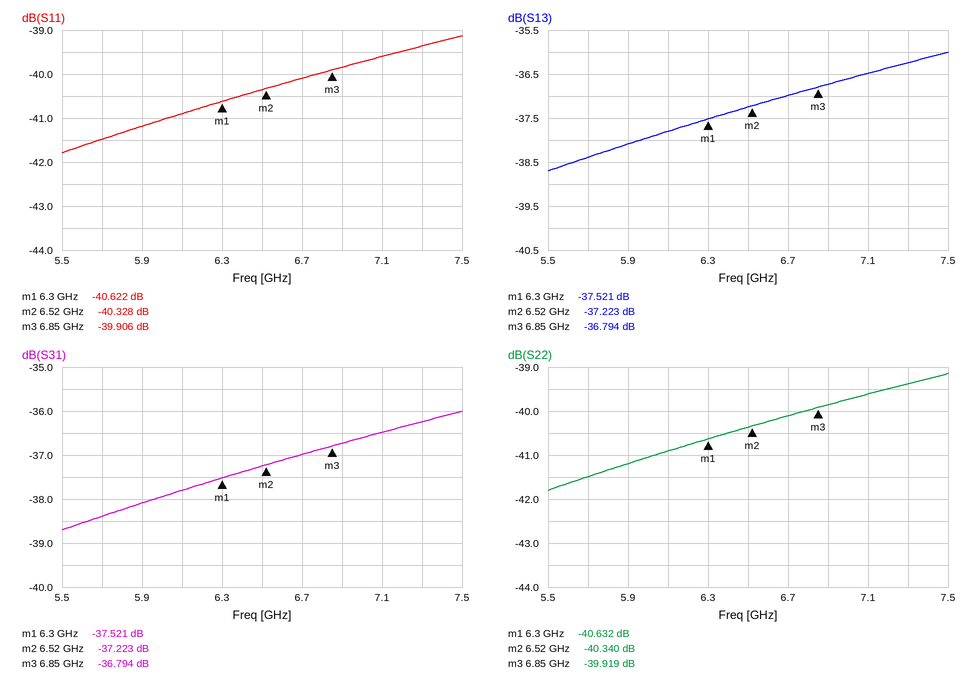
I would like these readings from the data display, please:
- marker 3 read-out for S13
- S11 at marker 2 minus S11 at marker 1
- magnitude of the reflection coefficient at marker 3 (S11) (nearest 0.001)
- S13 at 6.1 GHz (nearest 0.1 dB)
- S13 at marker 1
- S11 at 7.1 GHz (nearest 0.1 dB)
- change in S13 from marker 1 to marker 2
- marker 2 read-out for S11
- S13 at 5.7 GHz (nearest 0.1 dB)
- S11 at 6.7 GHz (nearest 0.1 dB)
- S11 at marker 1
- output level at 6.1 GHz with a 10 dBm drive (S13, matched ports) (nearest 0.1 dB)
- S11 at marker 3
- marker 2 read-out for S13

-36.794 dB
0.294 dB
0.010
-37.8 dB
-37.521 dB
-39.6 dB
0.298 dB
-40.328 dB
-38.4 dB
-40.1 dB
-40.622 dB
-27.8 dBm
-39.906 dB
-37.223 dB
